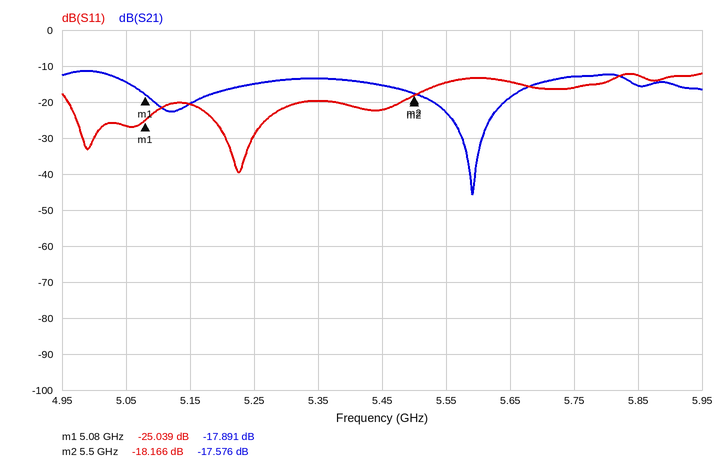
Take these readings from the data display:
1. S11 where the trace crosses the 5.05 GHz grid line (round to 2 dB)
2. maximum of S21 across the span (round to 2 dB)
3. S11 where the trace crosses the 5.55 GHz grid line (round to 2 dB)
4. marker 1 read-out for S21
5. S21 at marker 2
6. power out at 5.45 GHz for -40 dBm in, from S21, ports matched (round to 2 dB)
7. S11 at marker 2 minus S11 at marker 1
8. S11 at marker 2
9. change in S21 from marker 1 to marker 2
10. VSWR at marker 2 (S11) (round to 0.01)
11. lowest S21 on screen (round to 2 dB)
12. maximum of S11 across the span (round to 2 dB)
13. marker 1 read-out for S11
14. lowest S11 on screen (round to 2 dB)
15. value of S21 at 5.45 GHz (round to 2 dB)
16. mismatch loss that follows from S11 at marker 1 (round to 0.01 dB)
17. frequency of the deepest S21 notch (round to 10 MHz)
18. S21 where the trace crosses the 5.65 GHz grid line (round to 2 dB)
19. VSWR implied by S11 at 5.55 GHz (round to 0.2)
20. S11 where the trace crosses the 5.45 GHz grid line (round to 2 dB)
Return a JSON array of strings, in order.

["-26 dB", "-12 dB", "-14 dB", "-17.891 dB", "-17.576 dB", "-56 dBm", "6.873 dB", "-18.166 dB", "0.315 dB", "1.28", "-46 dB", "-12 dB", "-25.039 dB", "-40 dB", "-16 dB", "0.01 dB", "5.59 GHz", "-18 dB", "1.4", "-22 dB"]
